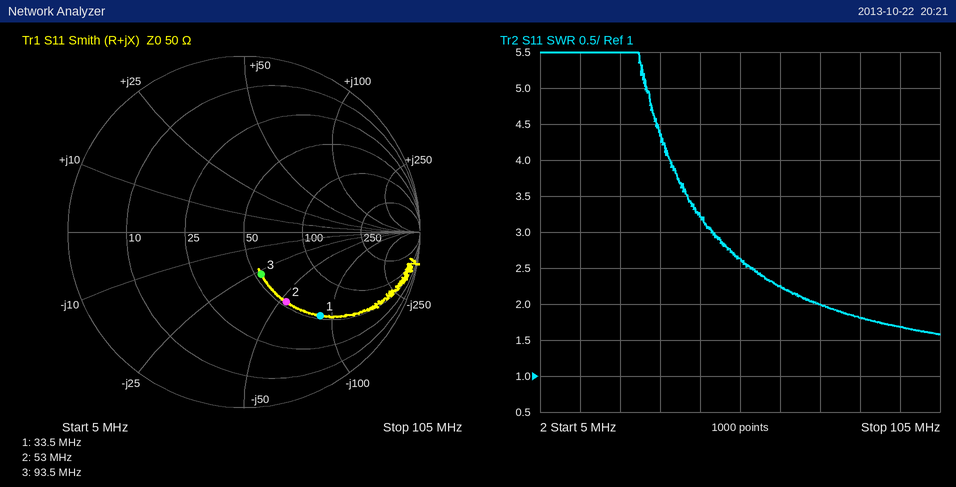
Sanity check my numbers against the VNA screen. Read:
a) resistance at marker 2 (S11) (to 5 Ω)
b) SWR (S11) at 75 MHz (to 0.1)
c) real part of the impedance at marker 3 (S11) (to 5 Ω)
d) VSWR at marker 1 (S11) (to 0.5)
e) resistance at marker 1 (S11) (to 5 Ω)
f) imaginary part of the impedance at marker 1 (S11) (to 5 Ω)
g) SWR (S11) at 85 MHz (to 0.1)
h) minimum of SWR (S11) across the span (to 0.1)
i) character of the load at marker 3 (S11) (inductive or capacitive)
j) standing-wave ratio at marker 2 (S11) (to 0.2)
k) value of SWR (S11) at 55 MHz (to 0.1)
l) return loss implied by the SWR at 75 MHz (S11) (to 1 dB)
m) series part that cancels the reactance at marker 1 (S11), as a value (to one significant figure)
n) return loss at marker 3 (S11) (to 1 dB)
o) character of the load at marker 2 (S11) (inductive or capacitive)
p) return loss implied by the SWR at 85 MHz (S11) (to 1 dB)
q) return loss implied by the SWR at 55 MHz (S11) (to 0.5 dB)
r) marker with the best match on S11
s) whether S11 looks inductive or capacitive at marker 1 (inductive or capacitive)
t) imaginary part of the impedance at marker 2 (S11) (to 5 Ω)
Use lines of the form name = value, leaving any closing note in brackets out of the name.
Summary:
resistance at marker 2 (S11) = 55 Ω
SWR (S11) at 75 MHz = 2.0
real part of the impedance at marker 3 (S11) = 55 Ω
VSWR at marker 1 (S11) = 4.5
resistance at marker 1 (S11) = 55 Ω
imaginary part of the impedance at marker 1 (S11) = -85 Ω
SWR (S11) at 85 MHz = 1.8
minimum of SWR (S11) across the span = 1.6
character of the load at marker 3 (S11) = capacitive
standing-wave ratio at marker 2 (S11) = 2.8
value of SWR (S11) at 55 MHz = 2.6
return loss implied by the SWR at 75 MHz (S11) = 10 dB
series part that cancels the reactance at marker 1 (S11), as a value = 400 nH
return loss at marker 3 (S11) = 12 dB
character of the load at marker 2 (S11) = capacitive
return loss implied by the SWR at 85 MHz (S11) = 11 dB
return loss implied by the SWR at 55 MHz (S11) = 7.0 dB
marker with the best match on S11 = marker 3
whether S11 looks inductive or capacitive at marker 1 = capacitive
imaginary part of the impedance at marker 2 (S11) = -55 Ω
